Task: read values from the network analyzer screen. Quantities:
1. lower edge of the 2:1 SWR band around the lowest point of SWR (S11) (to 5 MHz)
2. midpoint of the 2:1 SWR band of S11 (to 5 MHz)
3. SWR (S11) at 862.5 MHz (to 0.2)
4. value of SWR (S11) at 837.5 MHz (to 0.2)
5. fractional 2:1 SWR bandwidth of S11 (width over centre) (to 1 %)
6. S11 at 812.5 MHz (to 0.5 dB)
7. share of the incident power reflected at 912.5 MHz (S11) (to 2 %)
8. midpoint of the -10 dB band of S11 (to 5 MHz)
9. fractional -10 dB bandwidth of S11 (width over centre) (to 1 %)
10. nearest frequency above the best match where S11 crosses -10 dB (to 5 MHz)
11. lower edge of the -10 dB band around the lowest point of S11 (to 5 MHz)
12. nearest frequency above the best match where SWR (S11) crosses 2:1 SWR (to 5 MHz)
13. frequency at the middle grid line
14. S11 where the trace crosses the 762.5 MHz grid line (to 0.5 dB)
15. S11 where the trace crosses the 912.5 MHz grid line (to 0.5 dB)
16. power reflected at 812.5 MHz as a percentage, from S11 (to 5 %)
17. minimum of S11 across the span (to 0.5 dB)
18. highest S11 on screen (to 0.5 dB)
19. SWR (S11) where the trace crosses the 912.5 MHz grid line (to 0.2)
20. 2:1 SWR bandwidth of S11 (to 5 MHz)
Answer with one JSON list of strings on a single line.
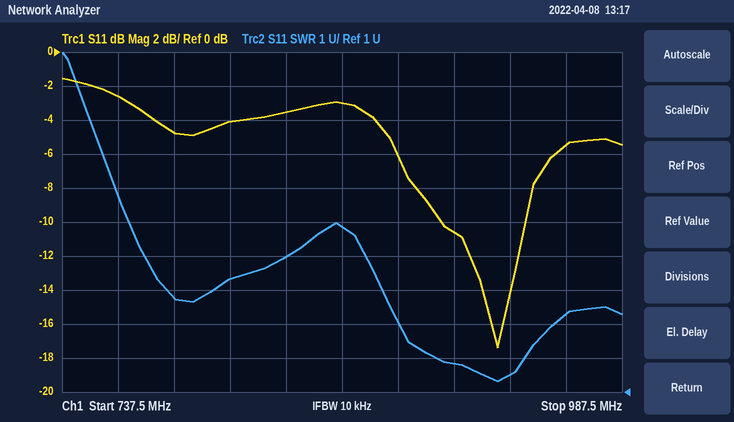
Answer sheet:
["905 MHz", "925 MHz", "5.8", "5.0", "4 %", "-4.0 dB", "8 %", "925 MHz", "4 %", "945 MHz", "905 MHz", "945 MHz", "862.5 MHz", "-2.5 dB", "-10.5 dB", "40 %", "-17.5 dB", "-1.5 dB", "1.8", "40 MHz"]
